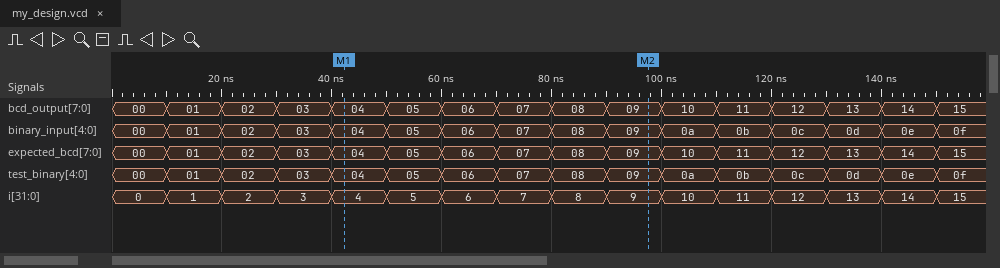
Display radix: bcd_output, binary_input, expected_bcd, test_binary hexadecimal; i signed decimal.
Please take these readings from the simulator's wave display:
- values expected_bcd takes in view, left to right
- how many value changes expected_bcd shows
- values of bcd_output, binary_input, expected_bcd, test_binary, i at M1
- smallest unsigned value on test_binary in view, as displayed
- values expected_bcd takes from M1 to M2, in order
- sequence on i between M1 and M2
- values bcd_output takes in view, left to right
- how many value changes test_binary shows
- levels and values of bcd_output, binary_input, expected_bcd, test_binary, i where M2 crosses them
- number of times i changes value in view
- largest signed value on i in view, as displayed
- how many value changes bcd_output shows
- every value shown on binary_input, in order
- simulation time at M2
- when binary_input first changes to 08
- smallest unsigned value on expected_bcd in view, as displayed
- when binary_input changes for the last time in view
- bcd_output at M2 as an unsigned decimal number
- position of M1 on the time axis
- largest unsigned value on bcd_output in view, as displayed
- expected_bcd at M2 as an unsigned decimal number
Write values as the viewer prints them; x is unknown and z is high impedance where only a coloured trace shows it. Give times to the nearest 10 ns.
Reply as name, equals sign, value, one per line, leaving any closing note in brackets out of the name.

values expected_bcd takes in view, left to right = 00, 01, 02, 03, 04, 05, 06, 07, 08, 09, 10, 11, 12, 13, 14, 15
how many value changes expected_bcd shows = 15
values of bcd_output, binary_input, expected_bcd, test_binary, i at M1 = bcd_output=04, binary_input=04, expected_bcd=04, test_binary=04, i=4
smallest unsigned value on test_binary in view, as displayed = 00
values expected_bcd takes from M1 to M2, in order = 04, 05, 06, 07, 08, 09
sequence on i between M1 and M2 = 4, 5, 6, 7, 8, 9
values bcd_output takes in view, left to right = 00, 01, 02, 03, 04, 05, 06, 07, 08, 09, 10, 11, 12, 13, 14, 15
how many value changes test_binary shows = 15
levels and values of bcd_output, binary_input, expected_bcd, test_binary, i where M2 crosses them = bcd_output=09, binary_input=09, expected_bcd=09, test_binary=09, i=9
number of times i changes value in view = 15
largest signed value on i in view, as displayed = 15
how many value changes bcd_output shows = 15
every value shown on binary_input, in order = 00, 01, 02, 03, 04, 05, 06, 07, 08, 09, 0a, 0b, 0c, 0d, 0e, 0f
simulation time at M2 = 100 ns
when binary_input first changes to 08 = 80 ns
smallest unsigned value on expected_bcd in view, as displayed = 00
when binary_input changes for the last time in view = 150 ns
bcd_output at M2 as an unsigned decimal number = 9
position of M1 on the time axis = 40 ns
largest unsigned value on bcd_output in view, as displayed = 15
expected_bcd at M2 as an unsigned decimal number = 9
